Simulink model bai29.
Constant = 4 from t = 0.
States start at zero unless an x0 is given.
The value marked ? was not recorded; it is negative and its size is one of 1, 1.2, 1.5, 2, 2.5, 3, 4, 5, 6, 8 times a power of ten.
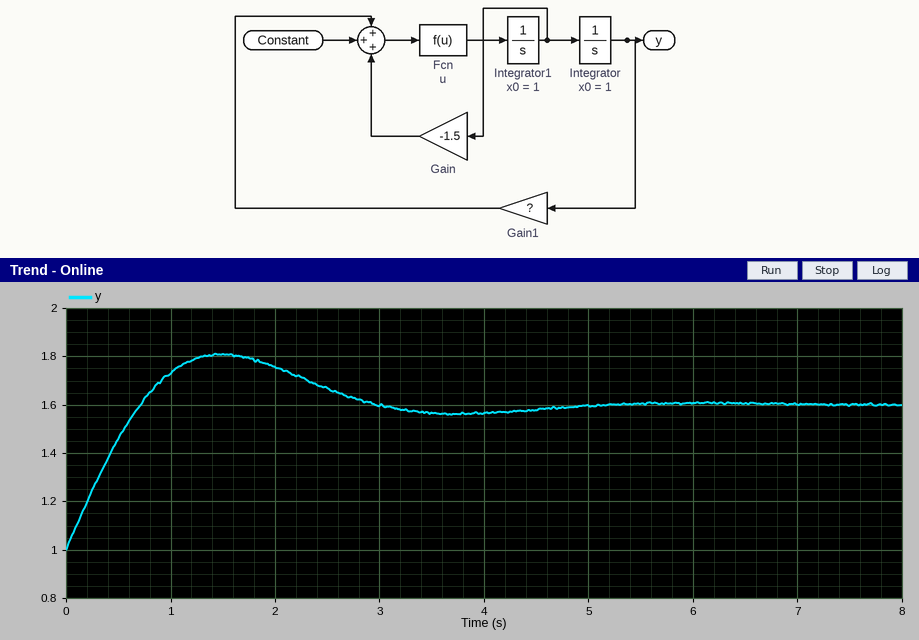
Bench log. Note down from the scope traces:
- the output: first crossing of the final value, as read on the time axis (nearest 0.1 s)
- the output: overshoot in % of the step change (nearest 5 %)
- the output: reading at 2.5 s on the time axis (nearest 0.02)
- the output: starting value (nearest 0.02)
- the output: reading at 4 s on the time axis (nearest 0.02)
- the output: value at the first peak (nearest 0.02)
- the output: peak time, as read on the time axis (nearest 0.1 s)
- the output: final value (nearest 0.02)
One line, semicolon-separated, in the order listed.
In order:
0.7 s; 35 %; 1.66; 1.00; 1.56; 1.80; 1.5 s; 1.60
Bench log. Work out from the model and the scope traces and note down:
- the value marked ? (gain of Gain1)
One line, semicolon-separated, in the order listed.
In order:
-2.5
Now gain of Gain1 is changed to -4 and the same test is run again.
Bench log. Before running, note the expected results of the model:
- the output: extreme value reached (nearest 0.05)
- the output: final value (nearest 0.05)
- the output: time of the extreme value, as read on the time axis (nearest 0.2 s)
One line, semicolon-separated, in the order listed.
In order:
1.30; 1.00; 0.6 s
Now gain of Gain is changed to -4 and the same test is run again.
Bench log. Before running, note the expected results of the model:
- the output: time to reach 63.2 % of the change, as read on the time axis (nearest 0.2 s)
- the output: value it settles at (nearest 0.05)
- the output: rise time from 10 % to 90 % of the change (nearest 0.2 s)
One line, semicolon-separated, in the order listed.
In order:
0.8 s; 1.60; 2.4 s
